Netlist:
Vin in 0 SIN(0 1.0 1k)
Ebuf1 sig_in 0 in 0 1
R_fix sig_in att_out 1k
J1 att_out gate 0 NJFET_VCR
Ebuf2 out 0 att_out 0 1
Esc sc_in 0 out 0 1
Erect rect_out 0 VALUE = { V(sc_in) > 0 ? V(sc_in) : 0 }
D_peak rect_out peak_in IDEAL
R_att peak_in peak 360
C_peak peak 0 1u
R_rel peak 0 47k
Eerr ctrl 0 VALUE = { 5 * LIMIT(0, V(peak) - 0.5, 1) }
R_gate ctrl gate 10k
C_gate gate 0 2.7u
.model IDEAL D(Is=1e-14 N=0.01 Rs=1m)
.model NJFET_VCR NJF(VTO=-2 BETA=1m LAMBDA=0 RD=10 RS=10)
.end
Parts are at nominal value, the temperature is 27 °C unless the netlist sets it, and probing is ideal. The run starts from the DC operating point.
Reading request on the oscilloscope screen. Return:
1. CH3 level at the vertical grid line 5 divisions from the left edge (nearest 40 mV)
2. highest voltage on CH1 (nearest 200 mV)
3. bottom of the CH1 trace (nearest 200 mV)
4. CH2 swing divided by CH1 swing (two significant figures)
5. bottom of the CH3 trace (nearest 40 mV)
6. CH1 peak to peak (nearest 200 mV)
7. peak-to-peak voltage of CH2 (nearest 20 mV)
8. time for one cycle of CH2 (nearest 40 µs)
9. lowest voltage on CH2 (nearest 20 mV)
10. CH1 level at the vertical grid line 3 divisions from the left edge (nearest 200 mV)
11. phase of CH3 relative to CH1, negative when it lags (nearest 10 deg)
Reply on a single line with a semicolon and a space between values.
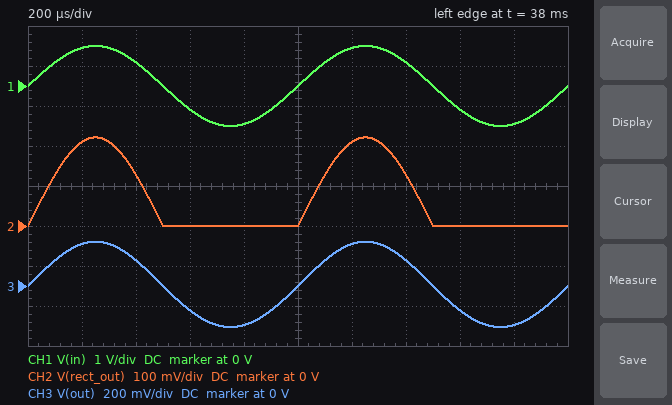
0 V; 1.0 V; -1.0 V; 0.11; -200 mV; 2.0 V; 220 mV; 1.00 ms; 0 V; -600 mV; 0 deg
